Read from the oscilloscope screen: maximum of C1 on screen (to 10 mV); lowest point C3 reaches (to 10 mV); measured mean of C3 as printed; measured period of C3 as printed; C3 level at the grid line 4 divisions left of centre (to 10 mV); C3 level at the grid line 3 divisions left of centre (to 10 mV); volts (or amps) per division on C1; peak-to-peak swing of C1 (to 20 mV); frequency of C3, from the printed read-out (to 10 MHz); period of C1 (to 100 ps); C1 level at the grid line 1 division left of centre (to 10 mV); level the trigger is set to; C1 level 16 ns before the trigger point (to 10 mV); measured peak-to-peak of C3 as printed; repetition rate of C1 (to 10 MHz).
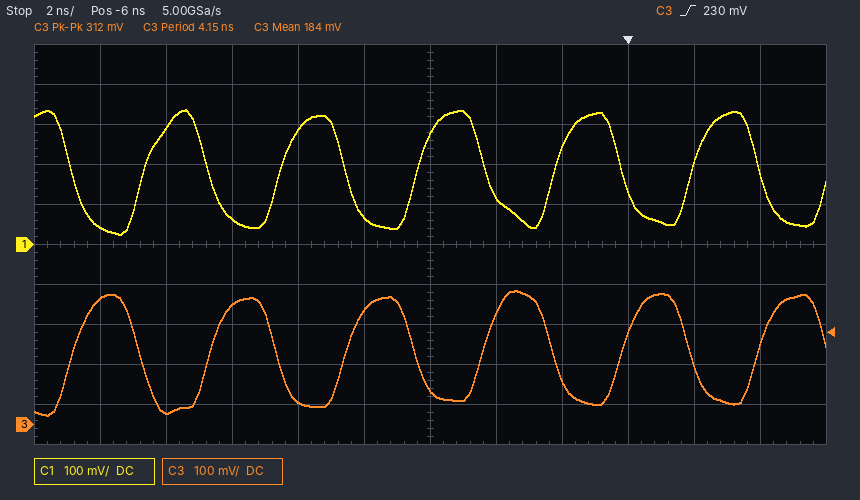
340 mV
20 mV
184 mV
4.15 ns
30 mV
300 mV
100 mV
320 mV
240 MHz
4.2 ns
70 mV
230 mV
40 mV
312 mV
240 MHz
